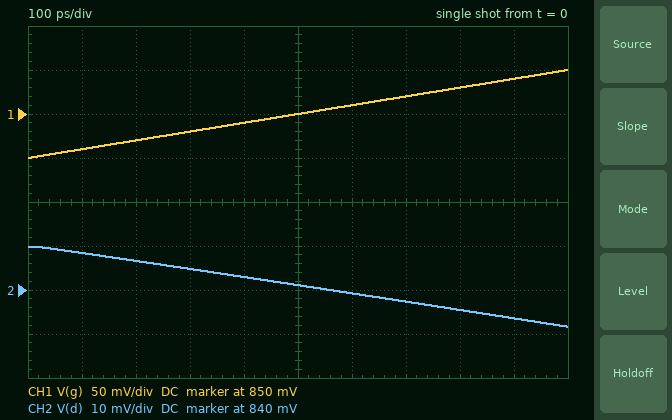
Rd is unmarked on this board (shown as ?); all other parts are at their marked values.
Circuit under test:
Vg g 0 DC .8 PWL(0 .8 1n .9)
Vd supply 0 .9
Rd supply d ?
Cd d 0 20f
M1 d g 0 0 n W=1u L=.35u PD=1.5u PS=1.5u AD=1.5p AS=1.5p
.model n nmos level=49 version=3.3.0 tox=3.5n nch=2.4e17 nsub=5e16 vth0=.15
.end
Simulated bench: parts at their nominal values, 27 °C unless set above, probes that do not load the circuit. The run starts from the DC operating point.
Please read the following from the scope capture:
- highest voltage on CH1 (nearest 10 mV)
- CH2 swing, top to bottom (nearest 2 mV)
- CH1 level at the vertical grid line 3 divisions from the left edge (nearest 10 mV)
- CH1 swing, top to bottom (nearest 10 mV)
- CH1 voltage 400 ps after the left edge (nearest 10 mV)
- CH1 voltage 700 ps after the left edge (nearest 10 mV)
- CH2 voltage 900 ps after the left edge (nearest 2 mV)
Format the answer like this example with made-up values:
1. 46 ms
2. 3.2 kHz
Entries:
1. 900 mV
2. 18 mV
3. 830 mV
4. 100 mV
5. 840 mV
6. 870 mV
7. 834 mV
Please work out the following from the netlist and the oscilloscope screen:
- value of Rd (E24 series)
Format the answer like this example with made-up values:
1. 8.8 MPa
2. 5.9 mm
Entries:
1. 680 Ω
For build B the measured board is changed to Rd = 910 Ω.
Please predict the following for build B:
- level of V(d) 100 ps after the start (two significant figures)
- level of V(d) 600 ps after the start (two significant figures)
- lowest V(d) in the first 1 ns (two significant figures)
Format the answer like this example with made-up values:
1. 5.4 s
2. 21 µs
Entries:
1. 830 mV
2. 820 mV
3. 810 mV
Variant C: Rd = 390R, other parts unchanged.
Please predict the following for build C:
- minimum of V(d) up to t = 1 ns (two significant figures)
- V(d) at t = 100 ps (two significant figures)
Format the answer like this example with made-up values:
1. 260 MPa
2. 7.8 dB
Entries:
1. 860 mV
2. 870 mV
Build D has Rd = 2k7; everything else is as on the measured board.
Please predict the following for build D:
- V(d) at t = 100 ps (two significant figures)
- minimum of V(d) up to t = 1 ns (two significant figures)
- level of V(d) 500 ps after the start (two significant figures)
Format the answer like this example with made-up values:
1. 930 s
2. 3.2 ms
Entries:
1. 700 mV
2. 640 mV
3. 670 mV
